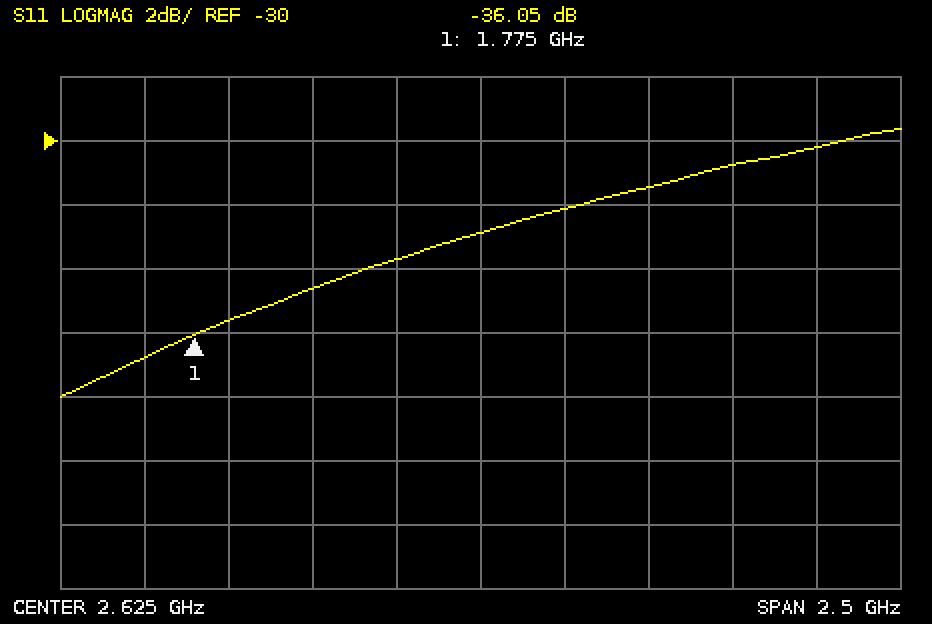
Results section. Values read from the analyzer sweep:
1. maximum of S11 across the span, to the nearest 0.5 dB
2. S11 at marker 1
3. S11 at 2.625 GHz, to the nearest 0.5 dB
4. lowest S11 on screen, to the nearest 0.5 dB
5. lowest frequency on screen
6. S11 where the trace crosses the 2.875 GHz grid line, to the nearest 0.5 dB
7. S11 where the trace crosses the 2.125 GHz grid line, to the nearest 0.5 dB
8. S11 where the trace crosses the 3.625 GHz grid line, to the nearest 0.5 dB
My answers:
-29.5 dB
-36.05 dB
-33.0 dB
-38.0 dB
1.375 GHz
-32.0 dB
-34.5 dB
-30.0 dB
